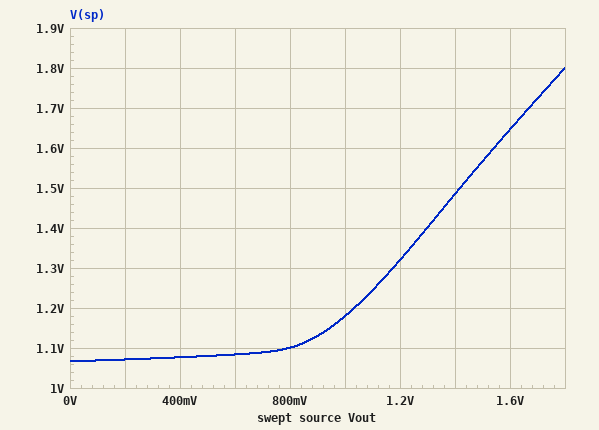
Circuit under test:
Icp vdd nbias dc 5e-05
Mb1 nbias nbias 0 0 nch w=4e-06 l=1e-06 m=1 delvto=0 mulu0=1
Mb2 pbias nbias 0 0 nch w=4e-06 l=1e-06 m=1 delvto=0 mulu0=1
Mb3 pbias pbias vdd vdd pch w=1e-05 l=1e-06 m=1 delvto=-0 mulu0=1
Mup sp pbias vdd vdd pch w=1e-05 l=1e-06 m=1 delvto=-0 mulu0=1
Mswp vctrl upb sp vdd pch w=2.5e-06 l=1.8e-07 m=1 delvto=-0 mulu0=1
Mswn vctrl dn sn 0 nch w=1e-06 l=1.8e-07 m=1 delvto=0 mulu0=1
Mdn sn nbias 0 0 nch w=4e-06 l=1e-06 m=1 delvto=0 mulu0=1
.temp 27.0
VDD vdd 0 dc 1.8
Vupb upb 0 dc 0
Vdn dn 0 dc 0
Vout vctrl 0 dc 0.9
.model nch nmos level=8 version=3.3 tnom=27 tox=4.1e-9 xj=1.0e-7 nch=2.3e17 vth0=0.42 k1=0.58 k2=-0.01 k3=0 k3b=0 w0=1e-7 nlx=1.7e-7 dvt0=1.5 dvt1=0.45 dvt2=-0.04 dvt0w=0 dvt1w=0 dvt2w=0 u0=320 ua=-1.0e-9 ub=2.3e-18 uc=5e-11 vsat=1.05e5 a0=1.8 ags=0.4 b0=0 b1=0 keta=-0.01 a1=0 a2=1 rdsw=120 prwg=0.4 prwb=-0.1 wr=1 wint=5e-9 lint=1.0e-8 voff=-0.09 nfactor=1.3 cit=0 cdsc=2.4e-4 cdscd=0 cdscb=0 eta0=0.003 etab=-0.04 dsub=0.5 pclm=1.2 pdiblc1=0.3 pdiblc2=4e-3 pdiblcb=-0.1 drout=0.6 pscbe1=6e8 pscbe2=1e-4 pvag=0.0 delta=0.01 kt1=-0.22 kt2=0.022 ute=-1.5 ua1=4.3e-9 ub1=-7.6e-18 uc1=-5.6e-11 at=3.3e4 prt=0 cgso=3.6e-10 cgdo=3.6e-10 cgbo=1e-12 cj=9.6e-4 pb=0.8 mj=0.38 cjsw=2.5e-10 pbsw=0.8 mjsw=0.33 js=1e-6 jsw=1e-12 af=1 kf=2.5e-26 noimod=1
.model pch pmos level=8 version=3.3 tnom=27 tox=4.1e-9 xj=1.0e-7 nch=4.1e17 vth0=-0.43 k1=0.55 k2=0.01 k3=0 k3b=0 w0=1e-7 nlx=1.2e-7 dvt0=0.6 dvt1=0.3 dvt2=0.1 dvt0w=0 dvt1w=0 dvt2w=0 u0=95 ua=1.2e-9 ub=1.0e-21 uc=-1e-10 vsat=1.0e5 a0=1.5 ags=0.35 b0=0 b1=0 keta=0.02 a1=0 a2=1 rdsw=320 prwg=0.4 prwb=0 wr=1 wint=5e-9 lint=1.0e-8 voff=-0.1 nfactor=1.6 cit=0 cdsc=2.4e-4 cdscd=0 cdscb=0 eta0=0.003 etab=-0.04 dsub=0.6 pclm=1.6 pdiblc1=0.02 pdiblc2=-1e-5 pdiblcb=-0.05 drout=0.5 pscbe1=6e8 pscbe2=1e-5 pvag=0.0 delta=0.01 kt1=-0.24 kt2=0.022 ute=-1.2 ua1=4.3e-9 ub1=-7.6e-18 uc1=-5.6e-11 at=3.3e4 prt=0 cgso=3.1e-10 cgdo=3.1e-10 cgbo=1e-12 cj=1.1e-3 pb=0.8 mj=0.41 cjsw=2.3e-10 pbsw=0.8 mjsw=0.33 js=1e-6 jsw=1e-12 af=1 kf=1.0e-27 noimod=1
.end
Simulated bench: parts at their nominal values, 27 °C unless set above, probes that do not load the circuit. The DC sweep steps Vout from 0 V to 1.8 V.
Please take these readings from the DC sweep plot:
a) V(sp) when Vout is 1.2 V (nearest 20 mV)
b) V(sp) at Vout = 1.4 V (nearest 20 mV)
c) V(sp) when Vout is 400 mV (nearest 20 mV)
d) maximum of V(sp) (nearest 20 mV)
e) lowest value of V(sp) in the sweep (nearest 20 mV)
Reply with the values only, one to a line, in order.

1.32 V
1.48 V
1.08 V
1.80 V
1.06 V
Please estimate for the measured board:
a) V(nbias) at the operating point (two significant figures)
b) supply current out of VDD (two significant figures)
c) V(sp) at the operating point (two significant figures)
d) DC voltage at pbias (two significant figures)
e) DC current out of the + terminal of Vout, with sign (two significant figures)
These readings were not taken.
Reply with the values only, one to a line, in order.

790 mV
150 µA
1.1 V
880 mV
-50 µA
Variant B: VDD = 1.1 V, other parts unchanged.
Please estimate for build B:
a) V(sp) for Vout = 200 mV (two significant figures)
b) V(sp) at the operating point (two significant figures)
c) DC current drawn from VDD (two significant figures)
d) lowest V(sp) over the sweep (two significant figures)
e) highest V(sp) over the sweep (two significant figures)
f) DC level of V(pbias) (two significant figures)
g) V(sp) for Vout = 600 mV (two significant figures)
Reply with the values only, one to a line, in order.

890 mV
980 mV
120 µA
880 mV
1.6 V
210 mV
900 mV
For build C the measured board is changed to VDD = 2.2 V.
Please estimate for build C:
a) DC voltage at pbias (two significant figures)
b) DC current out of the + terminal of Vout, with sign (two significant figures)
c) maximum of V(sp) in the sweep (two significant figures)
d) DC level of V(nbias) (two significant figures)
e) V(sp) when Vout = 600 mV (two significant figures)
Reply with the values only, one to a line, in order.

1.3 V
-51 µA
1.9 V
790 mV
1.2 V
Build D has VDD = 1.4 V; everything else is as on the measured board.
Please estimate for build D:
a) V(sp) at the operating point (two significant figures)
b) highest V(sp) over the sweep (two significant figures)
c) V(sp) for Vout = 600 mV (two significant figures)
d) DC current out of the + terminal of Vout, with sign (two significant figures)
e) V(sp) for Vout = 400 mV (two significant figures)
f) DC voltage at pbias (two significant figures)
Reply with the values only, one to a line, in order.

1.1 V
1.7 V
1.0 V
-46 µA
990 mV
490 mV
